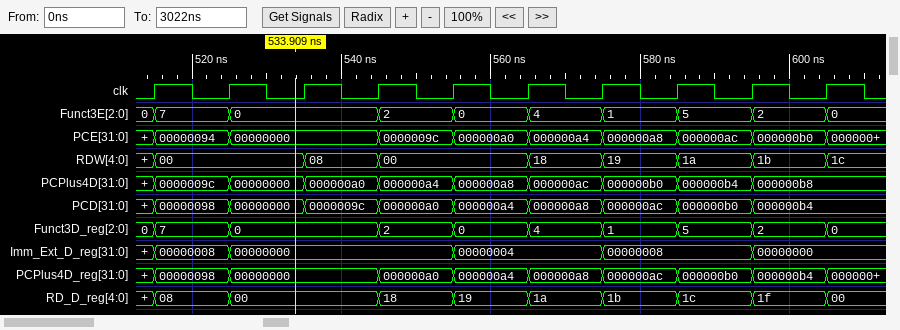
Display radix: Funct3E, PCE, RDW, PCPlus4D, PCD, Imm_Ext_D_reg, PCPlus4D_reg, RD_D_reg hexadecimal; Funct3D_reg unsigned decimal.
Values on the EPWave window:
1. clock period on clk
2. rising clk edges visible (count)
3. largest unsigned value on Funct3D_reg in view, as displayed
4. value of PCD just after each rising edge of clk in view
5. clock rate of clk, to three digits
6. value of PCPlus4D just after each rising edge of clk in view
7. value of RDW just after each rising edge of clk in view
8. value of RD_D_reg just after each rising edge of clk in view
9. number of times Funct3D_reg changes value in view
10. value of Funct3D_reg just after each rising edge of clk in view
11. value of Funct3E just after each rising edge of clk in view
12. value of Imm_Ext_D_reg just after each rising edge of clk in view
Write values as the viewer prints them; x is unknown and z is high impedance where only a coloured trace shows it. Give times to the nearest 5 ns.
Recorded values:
10 ns
10
7
00000098, 00000000, 0000009c, 000000a0, 000000a4, 000000a8, 000000ac, 000000b0, 000000b4, 000000b4
100 MHz
0000009c, 00000000, 000000a0, 000000a4, 000000a8, 000000ac, 000000b0, 000000b4, 000000b8, 000000b8
00, 00, 08, 00, 00, 18, 19, 1a, 1b, 1c
08, 00, 00, 18, 19, 1a, 1b, 1c, 1f, 00
9
7, 0, 0, 2, 0, 4, 1, 5, 2, 0
7, 0, 0, 2, 0, 4, 1, 5, 2, 0
00000008, 00000000, 00000000, 00000000, 00000004, 00000004, 00000008, 00000008, 00000000, 00000000
